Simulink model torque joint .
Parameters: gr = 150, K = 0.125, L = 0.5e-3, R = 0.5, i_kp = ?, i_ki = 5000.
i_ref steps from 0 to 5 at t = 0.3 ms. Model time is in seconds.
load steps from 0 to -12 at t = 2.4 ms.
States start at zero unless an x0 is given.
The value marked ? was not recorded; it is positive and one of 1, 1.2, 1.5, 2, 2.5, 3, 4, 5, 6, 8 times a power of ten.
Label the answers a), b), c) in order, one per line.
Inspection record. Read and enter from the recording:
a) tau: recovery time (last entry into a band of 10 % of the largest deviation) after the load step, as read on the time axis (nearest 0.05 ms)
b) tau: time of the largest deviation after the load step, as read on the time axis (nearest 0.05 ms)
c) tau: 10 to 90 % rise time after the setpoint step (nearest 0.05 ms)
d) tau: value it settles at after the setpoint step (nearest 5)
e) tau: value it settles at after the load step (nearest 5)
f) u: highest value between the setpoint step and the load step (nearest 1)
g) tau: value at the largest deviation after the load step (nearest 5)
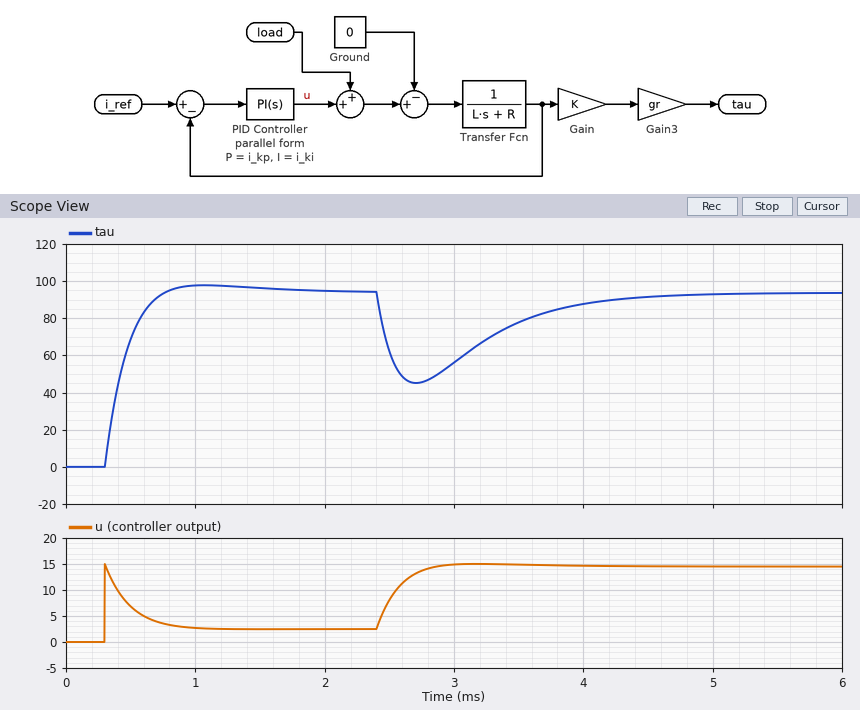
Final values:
a) 4.10 ms
b) 2.70 ms
c) 0.30 ms
d) 95
e) 95
f) 15
g) 45
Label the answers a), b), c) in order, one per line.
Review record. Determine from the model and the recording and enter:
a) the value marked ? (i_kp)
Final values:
a) 3
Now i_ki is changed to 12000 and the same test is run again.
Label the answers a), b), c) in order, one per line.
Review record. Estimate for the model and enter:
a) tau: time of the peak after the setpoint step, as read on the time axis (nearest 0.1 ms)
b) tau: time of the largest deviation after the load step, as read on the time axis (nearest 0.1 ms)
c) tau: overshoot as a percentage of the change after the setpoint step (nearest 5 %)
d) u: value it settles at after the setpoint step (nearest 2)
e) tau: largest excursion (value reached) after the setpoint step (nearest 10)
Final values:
a) 0.8 ms
b) 2.6 ms
c) 15 %
d) 2
e) 110
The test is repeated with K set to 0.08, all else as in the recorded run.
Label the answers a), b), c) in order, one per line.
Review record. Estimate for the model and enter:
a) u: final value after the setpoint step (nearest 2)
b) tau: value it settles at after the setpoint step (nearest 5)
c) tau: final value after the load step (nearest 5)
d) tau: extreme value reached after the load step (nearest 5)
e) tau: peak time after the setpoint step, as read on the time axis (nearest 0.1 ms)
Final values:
a) 2
b) 60
c) 60
d) 30
e) 1.1 ms
